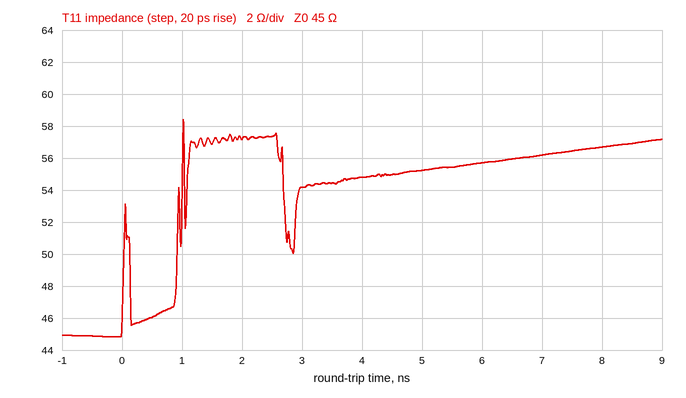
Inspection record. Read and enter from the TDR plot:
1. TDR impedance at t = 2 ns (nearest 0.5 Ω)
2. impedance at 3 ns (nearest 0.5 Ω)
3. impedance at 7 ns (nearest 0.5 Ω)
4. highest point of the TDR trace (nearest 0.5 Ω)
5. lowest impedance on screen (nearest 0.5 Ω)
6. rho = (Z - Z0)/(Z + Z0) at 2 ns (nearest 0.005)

57.0 Ω
54.0 Ω
56.0 Ω
58.5 Ω
45.0 Ω
+0.120
